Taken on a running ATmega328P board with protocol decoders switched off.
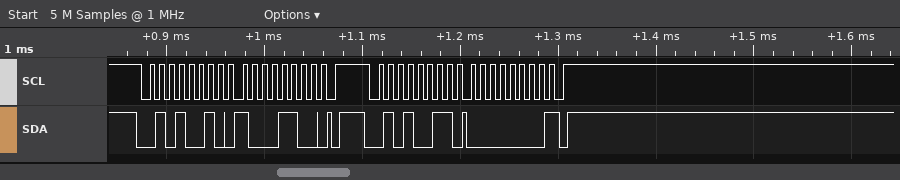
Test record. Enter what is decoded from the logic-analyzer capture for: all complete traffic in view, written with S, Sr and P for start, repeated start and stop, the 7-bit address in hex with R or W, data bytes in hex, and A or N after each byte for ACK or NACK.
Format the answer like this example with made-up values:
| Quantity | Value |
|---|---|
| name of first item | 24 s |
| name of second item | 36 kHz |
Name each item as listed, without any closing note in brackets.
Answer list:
| Quantity | Value |
|---|---|
| all complete traffic in view, written with S, Sr and P for start, repeated start and stop, the 7-bit address in hex with R or W, data bytes in hex, and A or N after each byte for ACK or NACK | S 29W A 8C A P S 29R A 00 N P |
